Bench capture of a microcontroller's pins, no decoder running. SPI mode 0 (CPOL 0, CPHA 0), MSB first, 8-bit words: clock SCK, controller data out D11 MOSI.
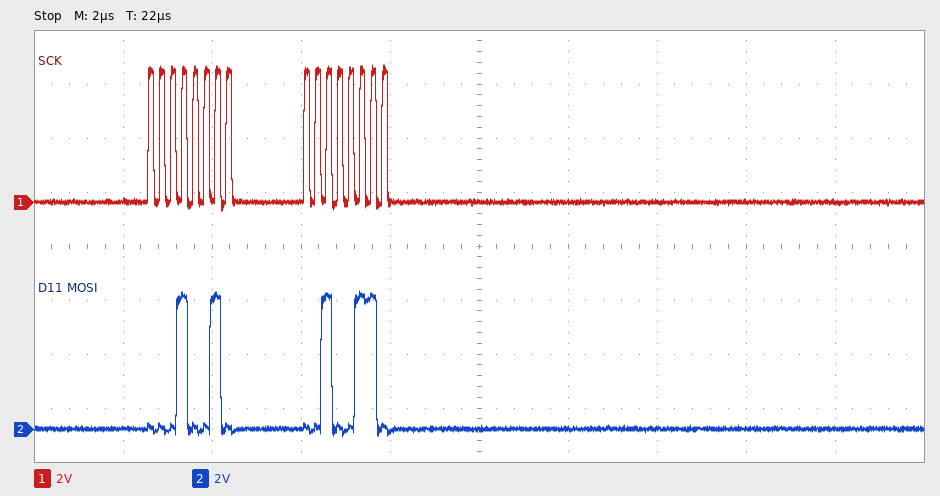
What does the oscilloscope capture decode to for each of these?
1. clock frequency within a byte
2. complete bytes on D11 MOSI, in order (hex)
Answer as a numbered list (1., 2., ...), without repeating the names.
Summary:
1. 4 MHz
2. 0x12 0x26
